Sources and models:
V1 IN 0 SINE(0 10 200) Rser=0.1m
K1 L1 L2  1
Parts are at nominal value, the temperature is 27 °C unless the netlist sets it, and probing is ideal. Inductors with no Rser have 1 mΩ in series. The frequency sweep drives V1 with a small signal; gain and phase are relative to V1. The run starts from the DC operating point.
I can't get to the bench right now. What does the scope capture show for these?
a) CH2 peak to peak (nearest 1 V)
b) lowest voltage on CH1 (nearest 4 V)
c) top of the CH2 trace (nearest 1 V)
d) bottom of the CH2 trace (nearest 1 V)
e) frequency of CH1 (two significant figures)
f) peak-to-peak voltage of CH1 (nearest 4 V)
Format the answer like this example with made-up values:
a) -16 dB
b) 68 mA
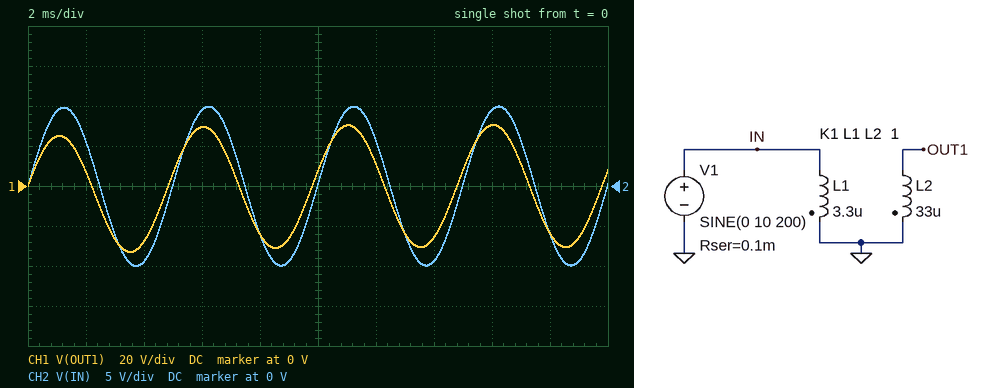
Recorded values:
a) 20 V
b) -32 V
c) 10 V
d) -10 V
e) 200 Hz
f) 64 V
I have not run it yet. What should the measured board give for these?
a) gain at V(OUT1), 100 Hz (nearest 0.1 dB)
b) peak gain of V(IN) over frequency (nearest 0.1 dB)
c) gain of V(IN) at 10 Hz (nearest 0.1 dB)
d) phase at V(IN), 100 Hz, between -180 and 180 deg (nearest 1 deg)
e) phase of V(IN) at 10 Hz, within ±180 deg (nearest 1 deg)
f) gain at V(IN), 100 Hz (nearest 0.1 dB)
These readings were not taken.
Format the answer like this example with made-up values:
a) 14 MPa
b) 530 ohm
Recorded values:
a) 8.9 dB
b) 0 dB
c) -0.8 dB
d) 2 deg
e) 1 deg
f) -0.2 dB
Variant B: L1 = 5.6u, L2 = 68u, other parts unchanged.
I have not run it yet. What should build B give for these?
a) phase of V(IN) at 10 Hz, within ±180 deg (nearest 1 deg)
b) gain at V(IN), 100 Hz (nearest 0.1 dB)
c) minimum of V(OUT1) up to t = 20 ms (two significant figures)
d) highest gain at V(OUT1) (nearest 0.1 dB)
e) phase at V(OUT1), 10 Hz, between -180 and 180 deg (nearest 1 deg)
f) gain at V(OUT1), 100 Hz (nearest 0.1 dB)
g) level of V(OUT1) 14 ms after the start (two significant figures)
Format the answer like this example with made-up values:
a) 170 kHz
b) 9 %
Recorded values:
a) 2 deg
b) -0.1 dB
c) -37 V
d) 10.8 dB
e) 72 deg
f) 10.4 dB
g) -31 V
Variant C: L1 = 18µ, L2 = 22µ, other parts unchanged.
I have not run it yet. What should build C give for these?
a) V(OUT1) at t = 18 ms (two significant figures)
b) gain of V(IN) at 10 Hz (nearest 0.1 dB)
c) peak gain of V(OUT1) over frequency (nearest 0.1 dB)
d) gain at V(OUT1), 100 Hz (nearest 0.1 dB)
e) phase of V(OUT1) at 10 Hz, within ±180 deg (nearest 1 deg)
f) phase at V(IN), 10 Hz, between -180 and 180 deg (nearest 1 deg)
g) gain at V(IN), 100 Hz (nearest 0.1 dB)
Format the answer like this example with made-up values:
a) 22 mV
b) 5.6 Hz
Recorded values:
a) -7.1 V
b) -0.4 dB
c) 0.9 dB
d) 0.8 dB
e) 44 deg
f) 3 deg
g) 0 dB
